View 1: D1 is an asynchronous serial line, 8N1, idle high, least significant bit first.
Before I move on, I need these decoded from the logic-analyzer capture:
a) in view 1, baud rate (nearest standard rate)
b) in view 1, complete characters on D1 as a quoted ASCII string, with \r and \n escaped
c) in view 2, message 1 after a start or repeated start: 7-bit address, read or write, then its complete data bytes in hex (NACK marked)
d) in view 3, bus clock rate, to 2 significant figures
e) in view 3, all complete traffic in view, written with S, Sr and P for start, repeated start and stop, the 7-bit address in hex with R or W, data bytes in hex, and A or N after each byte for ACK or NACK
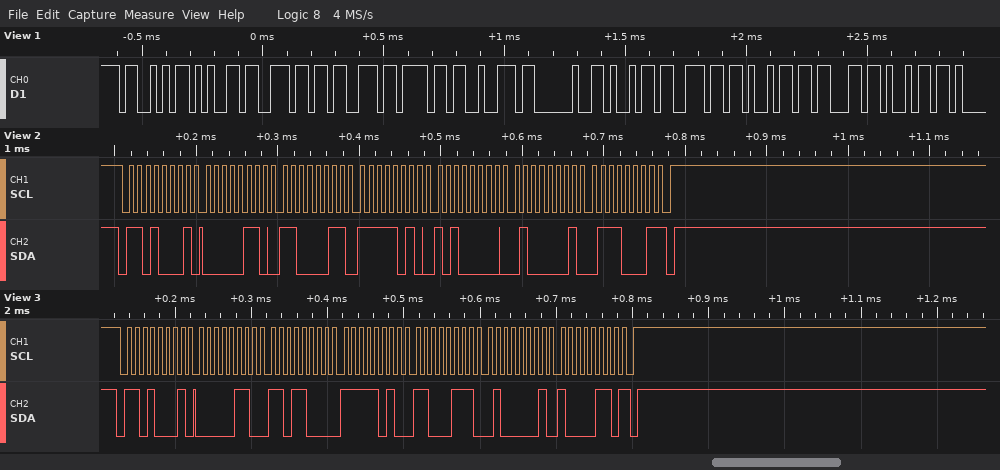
38400 baud
"Sensor inici"
0x68 read: 06 C3 FA A0 41 71 NACK
100 kHz
S 68R A 06 A D8 A FA A C7 A 41 A 86 N P
